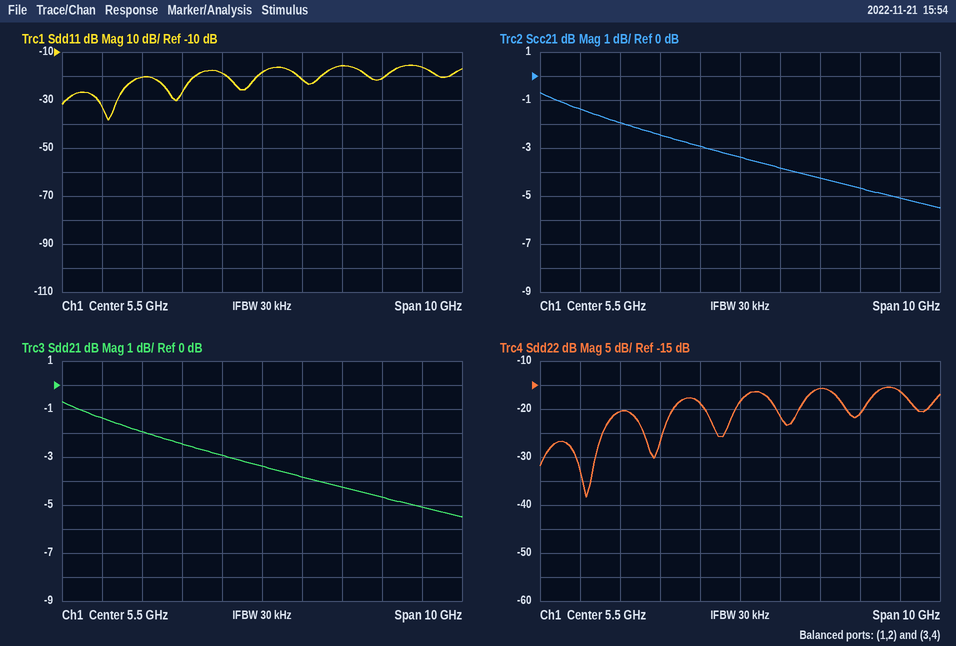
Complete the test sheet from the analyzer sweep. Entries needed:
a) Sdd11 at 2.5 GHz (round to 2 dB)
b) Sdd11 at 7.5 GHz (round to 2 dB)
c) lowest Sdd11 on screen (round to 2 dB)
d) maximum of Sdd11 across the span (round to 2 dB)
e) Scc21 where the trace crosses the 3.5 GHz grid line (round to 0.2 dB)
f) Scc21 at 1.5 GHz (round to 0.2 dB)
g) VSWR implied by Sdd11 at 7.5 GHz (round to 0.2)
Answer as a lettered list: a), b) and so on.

a) -20 dB
b) -16 dB
c) -38 dB
d) -16 dB
e) -2.4 dB
f) -1.4 dB
g) 1.4
